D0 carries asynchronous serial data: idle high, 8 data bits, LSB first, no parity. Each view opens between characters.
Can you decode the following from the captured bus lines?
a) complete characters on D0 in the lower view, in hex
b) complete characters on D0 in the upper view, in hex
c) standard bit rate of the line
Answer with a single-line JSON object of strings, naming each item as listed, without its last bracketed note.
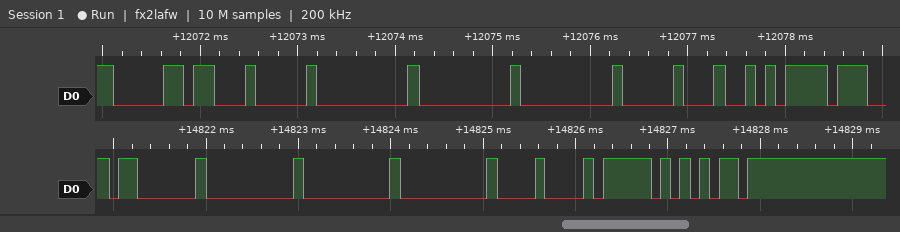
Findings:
{"complete characters on D0 in the lower view, in hex": "03, 00, 00, 00, 08, 5F, ED", "complete characters on D0 in the upper view, in hex": "B0, 04, 00, 00, 00, 10, EA", "standard bit rate of the line": "9600 baud"}
